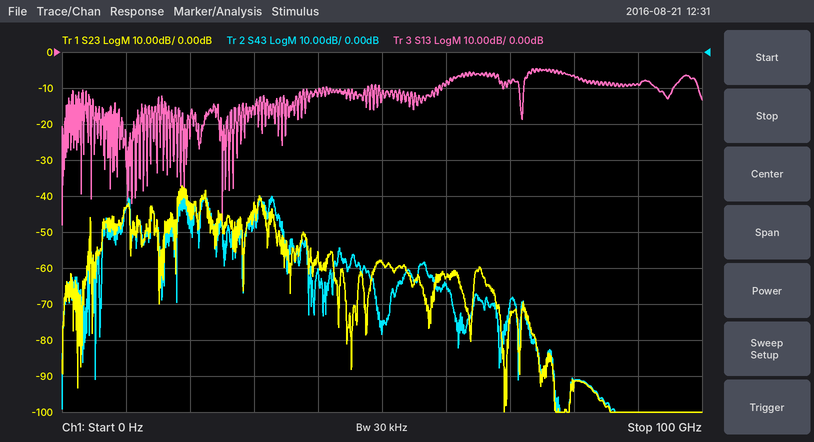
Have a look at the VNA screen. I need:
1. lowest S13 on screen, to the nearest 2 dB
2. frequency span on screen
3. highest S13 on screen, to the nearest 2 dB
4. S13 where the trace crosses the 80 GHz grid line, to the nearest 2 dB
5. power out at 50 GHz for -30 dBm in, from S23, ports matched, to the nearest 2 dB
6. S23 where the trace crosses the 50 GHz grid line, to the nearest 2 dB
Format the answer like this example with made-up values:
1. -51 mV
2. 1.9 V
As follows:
1. -48 dB
2. 100 GHz
3. -4 dB
4. -6 dB
5. -88 dBm
6. -58 dB
